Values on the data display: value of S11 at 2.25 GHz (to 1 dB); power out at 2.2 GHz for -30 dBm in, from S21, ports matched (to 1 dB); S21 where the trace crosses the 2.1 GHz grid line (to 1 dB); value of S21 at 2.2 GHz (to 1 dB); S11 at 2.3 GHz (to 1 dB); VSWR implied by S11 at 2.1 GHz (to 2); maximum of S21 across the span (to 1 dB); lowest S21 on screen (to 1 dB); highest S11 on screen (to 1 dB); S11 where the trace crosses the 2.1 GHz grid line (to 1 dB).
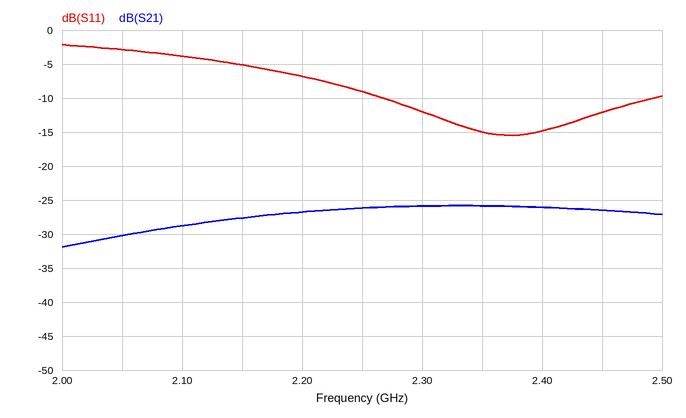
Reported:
-9 dB
-57 dBm
-29 dB
-27 dB
-12 dB
4
-26 dB
-32 dB
-2 dB
-4 dB
